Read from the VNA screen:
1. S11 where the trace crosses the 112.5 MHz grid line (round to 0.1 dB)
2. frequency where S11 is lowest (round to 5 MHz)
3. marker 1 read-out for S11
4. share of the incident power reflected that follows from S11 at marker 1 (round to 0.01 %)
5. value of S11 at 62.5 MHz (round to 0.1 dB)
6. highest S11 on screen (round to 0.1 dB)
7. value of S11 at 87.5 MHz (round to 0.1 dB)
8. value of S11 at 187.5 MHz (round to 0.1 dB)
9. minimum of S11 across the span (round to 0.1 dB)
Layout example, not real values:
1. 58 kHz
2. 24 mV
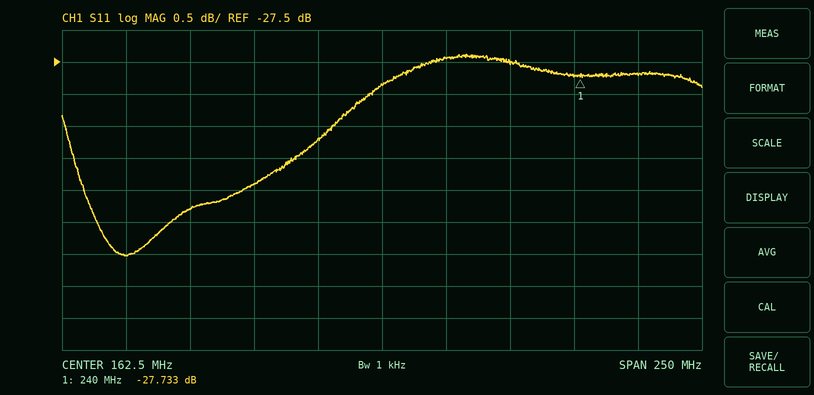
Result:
1. -29.4 dB
2. 60 MHz
3. -27.733 dB
4. 0.17 %
5. -30.5 dB
6. -27.4 dB
7. -29.8 dB
8. -27.4 dB
9. -30.5 dB
